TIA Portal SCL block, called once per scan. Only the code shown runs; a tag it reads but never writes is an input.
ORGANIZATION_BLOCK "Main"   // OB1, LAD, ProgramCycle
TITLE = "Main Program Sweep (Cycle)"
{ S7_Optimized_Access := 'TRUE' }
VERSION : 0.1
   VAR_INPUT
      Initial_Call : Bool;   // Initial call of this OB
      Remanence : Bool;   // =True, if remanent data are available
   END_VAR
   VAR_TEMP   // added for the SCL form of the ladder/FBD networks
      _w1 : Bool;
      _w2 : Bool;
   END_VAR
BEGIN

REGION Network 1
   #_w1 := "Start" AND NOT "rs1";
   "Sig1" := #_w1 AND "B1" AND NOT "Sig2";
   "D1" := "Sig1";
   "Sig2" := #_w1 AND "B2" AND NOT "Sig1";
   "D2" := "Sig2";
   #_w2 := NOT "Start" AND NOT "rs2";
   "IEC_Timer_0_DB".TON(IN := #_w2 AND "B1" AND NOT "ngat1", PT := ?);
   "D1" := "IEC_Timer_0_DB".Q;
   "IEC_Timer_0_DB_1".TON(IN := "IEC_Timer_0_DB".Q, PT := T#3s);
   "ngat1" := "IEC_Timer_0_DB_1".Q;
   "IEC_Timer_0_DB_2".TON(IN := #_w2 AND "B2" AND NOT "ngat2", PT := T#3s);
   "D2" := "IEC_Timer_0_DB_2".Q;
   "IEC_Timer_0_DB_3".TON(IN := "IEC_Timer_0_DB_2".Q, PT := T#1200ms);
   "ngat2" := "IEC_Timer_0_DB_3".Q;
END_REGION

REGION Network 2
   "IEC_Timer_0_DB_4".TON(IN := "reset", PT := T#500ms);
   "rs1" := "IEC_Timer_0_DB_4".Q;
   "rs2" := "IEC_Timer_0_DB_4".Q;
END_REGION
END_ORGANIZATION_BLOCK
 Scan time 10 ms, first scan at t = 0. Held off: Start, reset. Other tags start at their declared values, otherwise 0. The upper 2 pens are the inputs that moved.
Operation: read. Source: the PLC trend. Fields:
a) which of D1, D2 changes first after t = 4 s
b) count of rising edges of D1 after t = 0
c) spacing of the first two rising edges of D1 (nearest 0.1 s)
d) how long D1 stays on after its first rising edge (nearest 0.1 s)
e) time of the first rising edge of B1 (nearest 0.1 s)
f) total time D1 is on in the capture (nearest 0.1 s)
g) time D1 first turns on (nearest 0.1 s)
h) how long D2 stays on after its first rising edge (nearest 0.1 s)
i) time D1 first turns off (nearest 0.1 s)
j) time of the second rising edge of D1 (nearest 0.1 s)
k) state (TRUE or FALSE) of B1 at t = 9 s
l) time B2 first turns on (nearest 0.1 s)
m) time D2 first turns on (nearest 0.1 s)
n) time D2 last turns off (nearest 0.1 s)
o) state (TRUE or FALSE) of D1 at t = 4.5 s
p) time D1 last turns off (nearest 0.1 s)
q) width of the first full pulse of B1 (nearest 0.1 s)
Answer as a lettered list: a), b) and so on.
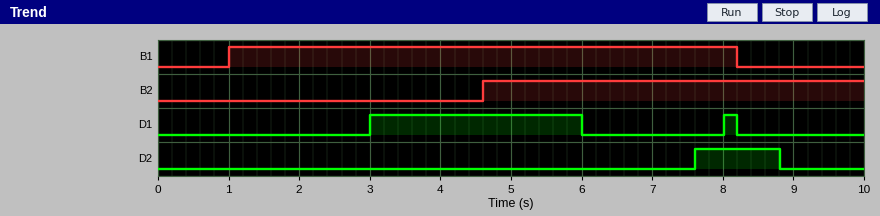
a) D1
b) 2
c) 5.0 s
d) 3.0 s
e) 1.0 s
f) 3.2 s
g) 3.0 s
h) 1.2 s
i) 6.0 s
j) 8.0 s
k) FALSE
l) 4.6 s
m) 7.6 s
n) 8.8 s
o) TRUE
p) 8.2 s
q) 7.2 s
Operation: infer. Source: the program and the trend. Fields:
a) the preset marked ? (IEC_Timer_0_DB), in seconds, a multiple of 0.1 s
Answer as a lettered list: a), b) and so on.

a) 2.0 s
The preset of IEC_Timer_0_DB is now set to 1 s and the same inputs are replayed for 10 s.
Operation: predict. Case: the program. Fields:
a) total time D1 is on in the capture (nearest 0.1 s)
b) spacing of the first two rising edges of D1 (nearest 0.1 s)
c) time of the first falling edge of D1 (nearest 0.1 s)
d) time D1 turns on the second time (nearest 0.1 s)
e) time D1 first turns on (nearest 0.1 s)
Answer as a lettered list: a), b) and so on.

a) 5.2 s
b) 4.0 s
c) 5.0 s
d) 6.0 s
e) 2.0 s
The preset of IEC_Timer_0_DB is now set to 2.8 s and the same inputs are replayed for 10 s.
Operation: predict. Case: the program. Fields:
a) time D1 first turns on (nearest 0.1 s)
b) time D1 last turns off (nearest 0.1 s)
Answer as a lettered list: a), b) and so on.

a) 3.8 s
b) 6.8 s
